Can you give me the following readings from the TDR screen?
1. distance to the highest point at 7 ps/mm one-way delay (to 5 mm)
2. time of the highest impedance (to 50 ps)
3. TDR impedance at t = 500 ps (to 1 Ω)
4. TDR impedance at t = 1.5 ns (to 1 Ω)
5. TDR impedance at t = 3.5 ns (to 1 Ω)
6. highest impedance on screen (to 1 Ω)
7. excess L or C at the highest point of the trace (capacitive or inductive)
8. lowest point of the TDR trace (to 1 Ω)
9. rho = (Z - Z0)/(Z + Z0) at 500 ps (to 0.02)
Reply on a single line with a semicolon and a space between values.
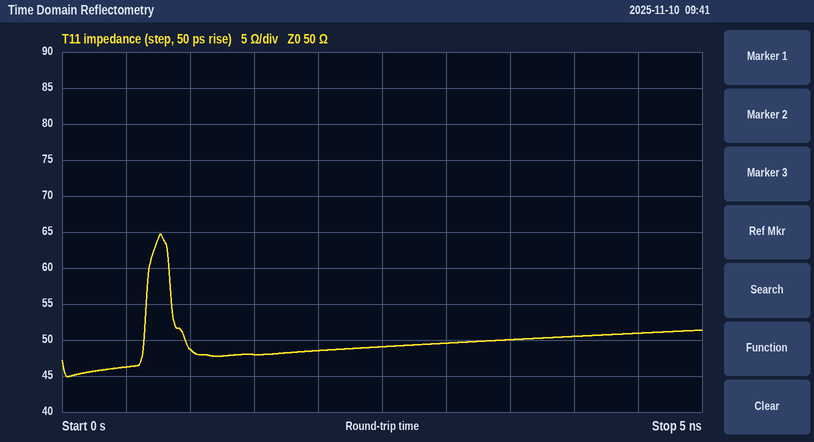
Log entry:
55 mm; 750 ps; 46 Ω; 48 Ω; 50 Ω; 65 Ω; inductive; 45 Ω; -0.04
